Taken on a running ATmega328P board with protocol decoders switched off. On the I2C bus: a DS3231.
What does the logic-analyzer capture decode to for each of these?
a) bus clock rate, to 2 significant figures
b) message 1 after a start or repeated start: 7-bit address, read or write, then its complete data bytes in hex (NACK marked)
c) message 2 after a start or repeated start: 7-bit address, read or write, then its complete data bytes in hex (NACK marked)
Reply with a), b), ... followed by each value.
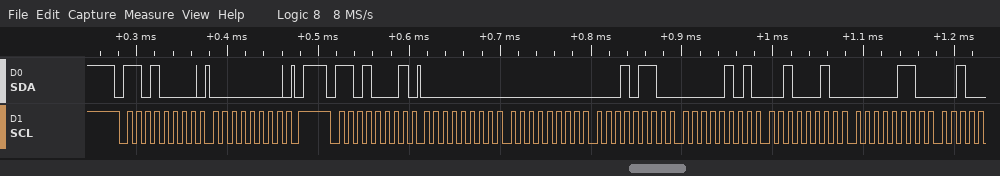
a) 100 kHz
b) 0x68 write: 00
c) 0x68 read: 00 00 16 05 22 06
